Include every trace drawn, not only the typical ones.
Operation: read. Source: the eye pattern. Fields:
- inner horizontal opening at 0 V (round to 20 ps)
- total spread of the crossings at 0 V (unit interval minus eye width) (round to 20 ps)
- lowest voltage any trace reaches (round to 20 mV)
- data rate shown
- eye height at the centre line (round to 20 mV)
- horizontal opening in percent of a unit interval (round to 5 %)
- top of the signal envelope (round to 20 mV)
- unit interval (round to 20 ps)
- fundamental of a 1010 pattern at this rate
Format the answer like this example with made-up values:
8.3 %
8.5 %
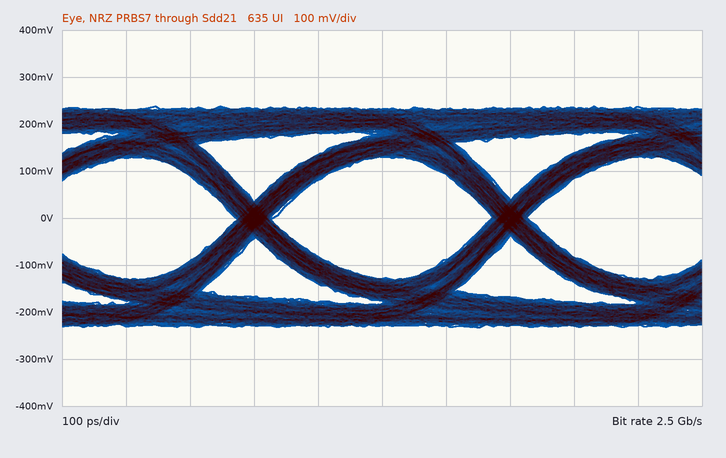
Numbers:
340 ps
60 ps
-240 mV
2.5 Gb/s
260 mV
85 %
240 mV
400 ps
1.25 GHz
